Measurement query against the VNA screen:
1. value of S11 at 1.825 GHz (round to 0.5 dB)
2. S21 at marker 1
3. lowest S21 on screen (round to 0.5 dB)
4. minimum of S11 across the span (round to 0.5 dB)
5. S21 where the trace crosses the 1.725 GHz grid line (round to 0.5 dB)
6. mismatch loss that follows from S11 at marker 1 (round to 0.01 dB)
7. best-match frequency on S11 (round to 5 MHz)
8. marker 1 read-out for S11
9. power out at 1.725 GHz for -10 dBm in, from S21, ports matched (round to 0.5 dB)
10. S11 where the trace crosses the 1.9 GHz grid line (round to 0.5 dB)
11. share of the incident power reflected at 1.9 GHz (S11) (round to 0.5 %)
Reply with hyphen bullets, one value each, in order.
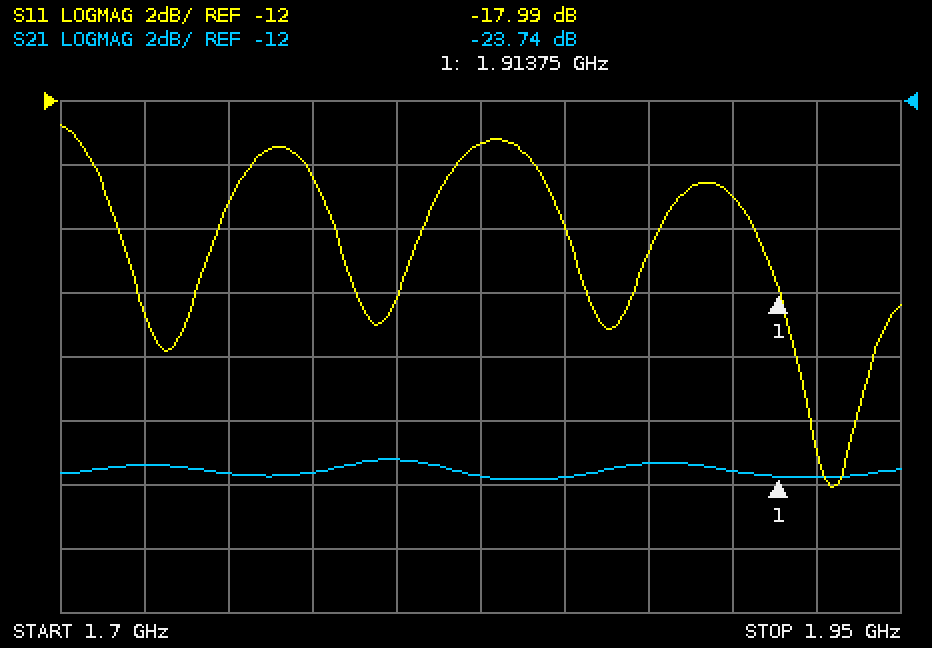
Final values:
- -13.5 dB
- -23.74 dB
- -24.0 dB
- -24.0 dB
- -23.5 dB
- 0.07 dB
- 1.930 GHz
- -17.99 dB
- -33.5 dBm
- -15.0 dB
- 3.0 %
